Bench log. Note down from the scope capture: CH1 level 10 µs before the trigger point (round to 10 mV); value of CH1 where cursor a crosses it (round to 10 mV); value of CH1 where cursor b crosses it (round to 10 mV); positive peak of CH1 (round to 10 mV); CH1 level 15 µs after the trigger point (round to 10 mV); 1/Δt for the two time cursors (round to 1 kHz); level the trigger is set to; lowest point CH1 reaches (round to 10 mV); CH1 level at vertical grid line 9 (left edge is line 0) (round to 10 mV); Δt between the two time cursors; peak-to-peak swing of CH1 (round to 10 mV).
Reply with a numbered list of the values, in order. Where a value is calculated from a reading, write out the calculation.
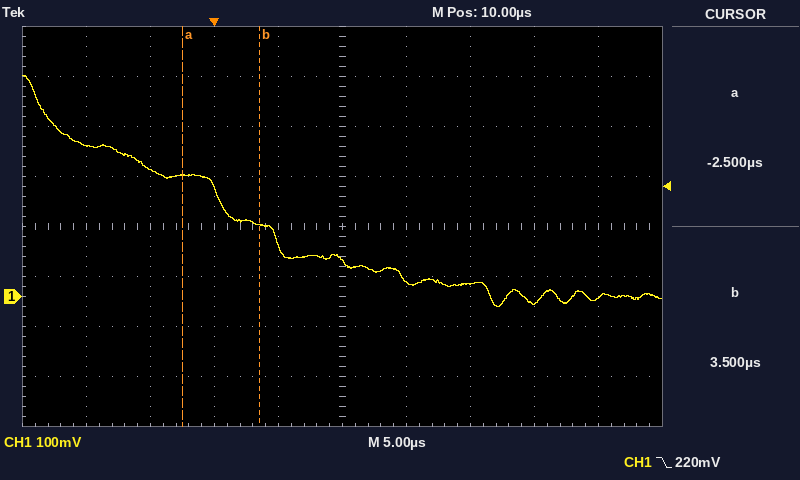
1. 300 mV
2. 240 mV
3. 140 mV
4. 440 mV
5. 30 mV
6. 1 / 6.0 µs ≈ 167 kHz
7. 220 mV
8. -20 mV
9. 0 mV
10. 3.5 µs − (-2.5 µs) = 6.0 µs
11. 440 mV − (-20 mV) = 460 mV
